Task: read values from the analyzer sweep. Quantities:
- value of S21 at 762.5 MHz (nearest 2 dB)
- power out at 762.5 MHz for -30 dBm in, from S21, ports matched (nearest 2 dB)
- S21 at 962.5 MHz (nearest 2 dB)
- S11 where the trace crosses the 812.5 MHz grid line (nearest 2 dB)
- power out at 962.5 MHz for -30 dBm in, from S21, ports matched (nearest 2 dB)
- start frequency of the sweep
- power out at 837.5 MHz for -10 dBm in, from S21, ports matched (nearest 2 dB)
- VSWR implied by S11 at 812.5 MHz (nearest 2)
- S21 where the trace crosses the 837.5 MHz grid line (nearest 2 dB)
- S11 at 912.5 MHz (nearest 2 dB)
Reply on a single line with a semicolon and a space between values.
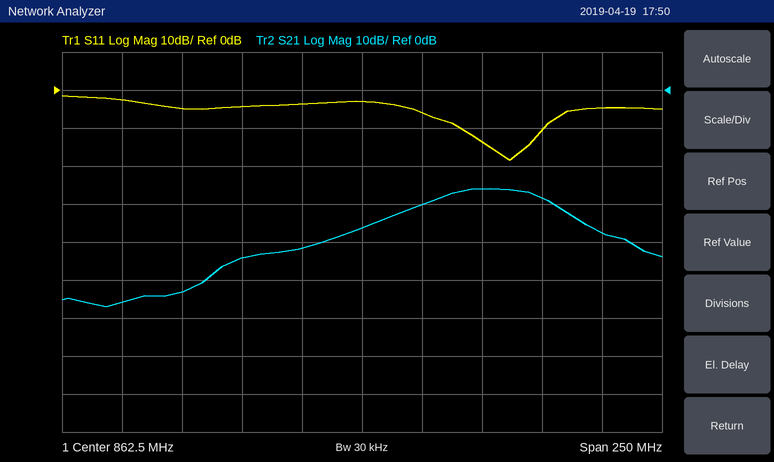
-56 dB; -86 dBm; -38 dB; -4 dB; -68 dBm; 737.5 MHz; -52 dBm; 4; -42 dB; -14 dB
